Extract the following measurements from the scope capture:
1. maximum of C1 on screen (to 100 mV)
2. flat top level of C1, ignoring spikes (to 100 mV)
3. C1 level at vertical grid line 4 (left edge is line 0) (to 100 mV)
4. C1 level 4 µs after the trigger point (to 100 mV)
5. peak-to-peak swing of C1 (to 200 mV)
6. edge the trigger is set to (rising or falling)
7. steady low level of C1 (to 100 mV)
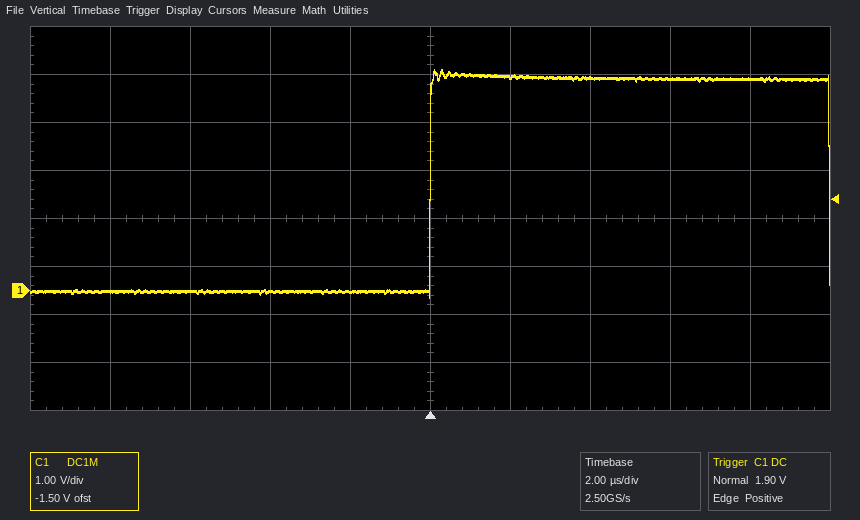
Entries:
4.6 V
4.4 V
0.0 V
4.4 V
4.8 V
rising
0.0 V
